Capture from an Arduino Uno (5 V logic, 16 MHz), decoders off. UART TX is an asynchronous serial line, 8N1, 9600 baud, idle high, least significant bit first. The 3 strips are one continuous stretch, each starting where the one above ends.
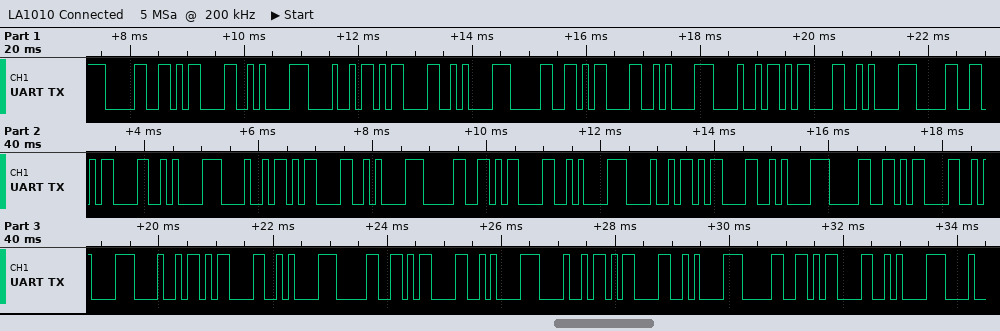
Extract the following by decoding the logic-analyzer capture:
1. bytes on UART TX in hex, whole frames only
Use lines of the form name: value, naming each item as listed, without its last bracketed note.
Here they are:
bytes on UART TX in hex, whole frames only: 30 0D 0A 48 0D 0A 30 0D 0A 48 0D 0A 30 0D 0A 48 0D 0A 30 0D 0A 48 0D 0A 30 0D 0A 48 0D 0A 30 0D 0A 48 0D 0A 30 0D 0A
